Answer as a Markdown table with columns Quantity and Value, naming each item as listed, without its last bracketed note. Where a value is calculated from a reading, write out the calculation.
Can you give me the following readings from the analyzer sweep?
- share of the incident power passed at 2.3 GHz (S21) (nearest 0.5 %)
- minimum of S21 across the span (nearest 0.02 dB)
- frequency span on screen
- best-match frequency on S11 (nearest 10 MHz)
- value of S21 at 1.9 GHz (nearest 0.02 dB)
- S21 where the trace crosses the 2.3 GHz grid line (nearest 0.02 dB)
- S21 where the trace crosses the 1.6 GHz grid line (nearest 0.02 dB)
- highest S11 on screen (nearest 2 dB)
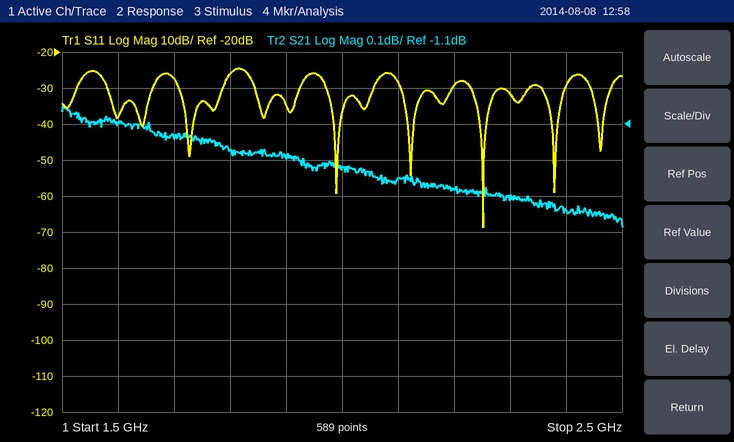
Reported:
| Quantity | Value |
|---|---|
| share of the incident power passed at 2.3 GHz (S21) | 10^(-1.3/10) ≈ 74.1 %, so 74.0 % to the nearest 0.5 % |
| minimum of S21 across the span | -1.38 dB |
| frequency span on screen | 1 GHz |
| best-match frequency on S11 | 2.25 GHz |
| value of S21 at 1.9 GHz | -1.20 dB |
| S21 where the trace crosses the 2.3 GHz grid line | -1.30 dB |
| S21 where the trace crosses the 1.6 GHz grid line | -1.10 dB |
| highest S11 on screen | -24 dB |
